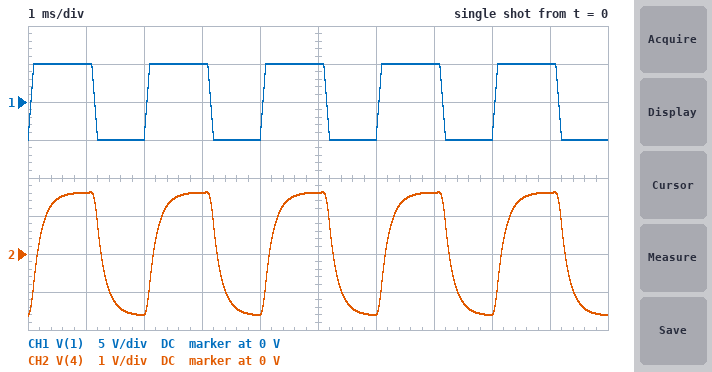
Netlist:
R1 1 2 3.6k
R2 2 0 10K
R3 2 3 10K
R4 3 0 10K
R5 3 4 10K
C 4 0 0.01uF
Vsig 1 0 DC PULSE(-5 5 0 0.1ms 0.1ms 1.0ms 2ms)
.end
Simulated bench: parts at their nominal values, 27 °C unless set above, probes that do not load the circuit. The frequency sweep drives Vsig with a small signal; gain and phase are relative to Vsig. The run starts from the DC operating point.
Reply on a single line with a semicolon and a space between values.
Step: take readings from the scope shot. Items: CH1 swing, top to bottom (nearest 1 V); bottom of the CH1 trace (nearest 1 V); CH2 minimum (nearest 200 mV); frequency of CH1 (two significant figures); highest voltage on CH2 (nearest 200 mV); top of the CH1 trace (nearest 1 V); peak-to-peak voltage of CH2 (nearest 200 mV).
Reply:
10 V; -5 V; -1.6 V; 500 Hz; 1.6 V; 5 V; 3.2 V
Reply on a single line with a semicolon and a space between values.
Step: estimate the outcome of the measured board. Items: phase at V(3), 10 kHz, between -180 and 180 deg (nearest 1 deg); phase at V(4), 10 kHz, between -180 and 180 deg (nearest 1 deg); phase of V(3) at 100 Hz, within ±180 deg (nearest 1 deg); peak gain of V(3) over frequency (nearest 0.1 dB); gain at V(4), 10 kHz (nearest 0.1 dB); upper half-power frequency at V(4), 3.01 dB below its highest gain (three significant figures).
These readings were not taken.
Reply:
-3 deg; -84 deg; -2 deg; -9.8 dB; -29.6 dB; 1.02 kHz
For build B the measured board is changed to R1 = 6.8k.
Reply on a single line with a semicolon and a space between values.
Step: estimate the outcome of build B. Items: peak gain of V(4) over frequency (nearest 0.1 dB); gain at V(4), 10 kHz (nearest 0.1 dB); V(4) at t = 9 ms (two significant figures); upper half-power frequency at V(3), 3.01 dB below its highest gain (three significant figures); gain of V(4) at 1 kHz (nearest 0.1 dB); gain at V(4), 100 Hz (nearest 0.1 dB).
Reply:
-12.1 dB; -32.1 dB; 1.2 V; 2.23 kHz; -15.1 dB; -12.2 dB
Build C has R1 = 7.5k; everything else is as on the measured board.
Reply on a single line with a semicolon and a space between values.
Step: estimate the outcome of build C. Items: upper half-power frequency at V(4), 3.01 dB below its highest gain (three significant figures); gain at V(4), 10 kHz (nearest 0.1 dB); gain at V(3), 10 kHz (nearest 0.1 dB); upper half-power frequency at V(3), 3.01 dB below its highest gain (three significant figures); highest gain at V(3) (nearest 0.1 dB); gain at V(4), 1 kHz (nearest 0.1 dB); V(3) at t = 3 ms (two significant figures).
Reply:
1.00 kHz; -32.6 dB; -16.5 dB; 2.20 kHz; -12.6 dB; -15.6 dB; 1.2 V
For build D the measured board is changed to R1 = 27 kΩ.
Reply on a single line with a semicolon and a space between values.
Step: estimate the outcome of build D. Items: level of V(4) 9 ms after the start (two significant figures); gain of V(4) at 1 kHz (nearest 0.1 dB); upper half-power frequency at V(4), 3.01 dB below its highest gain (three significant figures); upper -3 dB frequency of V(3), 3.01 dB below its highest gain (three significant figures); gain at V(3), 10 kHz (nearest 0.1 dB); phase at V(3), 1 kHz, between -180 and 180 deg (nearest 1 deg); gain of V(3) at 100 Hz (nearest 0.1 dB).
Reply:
490 mV; -23.2 dB; 974 Hz; 1.95 kHz; -24.3 dB; -14 deg; -20.1 dB
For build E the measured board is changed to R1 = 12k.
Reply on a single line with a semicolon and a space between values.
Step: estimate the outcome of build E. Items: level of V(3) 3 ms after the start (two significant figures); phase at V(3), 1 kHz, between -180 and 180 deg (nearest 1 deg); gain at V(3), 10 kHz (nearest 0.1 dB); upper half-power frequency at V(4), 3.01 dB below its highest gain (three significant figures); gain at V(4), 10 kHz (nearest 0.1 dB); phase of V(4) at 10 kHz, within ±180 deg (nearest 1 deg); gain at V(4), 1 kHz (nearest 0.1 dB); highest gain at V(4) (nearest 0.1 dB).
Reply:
890 mV; -13 deg; -19.0 dB; 990 Hz; -35.1 dB; -84 deg; -18.0 dB; -15.0 dB
